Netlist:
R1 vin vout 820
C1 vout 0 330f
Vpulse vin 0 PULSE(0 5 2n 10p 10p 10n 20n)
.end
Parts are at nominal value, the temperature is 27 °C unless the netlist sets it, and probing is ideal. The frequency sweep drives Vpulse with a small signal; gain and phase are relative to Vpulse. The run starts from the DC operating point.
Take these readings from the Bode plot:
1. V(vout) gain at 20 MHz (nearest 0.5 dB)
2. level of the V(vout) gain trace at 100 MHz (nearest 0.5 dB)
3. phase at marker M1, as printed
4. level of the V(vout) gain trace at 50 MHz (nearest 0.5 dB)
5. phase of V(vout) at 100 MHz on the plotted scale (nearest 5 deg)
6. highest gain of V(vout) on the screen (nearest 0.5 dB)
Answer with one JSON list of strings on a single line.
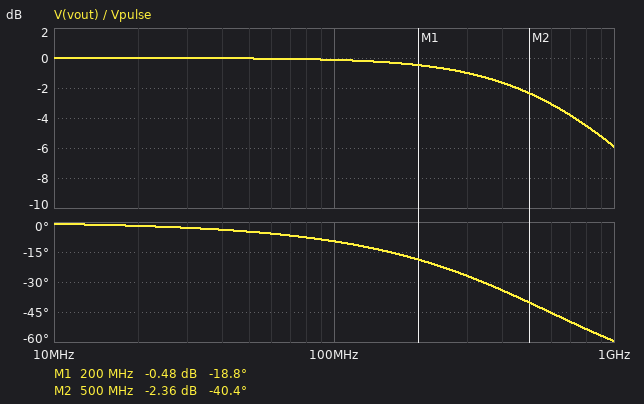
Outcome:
["0 dB", "0 dB", "-18.8 deg", "0 dB", "-10 deg", "0 dB"]
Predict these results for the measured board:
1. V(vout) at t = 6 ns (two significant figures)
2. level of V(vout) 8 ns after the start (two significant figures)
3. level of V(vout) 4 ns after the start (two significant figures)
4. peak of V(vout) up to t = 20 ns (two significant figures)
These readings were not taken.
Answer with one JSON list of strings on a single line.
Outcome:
["5.0 V", "5.0 V", "5.0 V", "5.0 V"]
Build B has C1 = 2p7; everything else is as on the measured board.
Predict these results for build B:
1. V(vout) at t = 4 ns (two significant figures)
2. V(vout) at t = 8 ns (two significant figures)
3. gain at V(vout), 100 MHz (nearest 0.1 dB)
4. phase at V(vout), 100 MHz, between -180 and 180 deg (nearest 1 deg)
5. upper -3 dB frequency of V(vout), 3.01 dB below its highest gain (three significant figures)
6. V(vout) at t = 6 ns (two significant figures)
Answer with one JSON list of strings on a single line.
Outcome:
["3.0 V", "4.7 V", "-4.7 dB", "-54 deg", "71.9 MHz", "4.2 V"]
